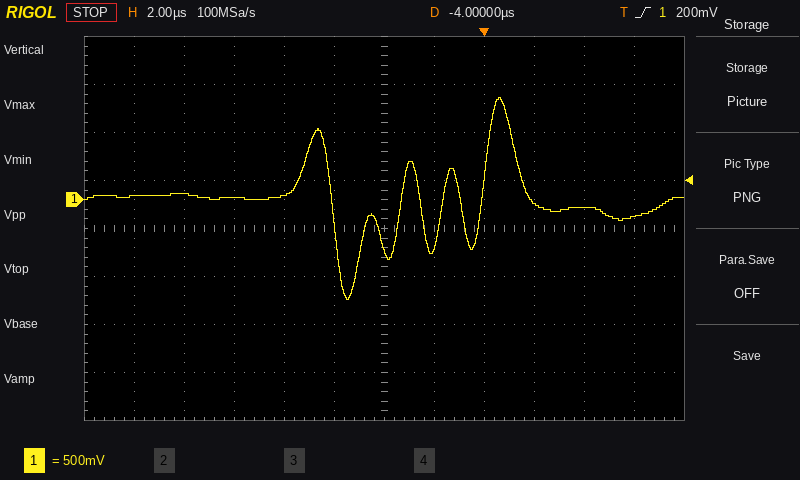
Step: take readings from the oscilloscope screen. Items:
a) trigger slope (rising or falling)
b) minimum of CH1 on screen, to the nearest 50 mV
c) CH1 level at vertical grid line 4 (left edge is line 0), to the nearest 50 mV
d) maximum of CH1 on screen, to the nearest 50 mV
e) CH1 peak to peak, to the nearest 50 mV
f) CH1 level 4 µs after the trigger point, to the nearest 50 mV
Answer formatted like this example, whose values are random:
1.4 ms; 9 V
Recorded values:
rising; -1.05 V; 50 mV; 1.05 V; 2.10 V; -100 mV
